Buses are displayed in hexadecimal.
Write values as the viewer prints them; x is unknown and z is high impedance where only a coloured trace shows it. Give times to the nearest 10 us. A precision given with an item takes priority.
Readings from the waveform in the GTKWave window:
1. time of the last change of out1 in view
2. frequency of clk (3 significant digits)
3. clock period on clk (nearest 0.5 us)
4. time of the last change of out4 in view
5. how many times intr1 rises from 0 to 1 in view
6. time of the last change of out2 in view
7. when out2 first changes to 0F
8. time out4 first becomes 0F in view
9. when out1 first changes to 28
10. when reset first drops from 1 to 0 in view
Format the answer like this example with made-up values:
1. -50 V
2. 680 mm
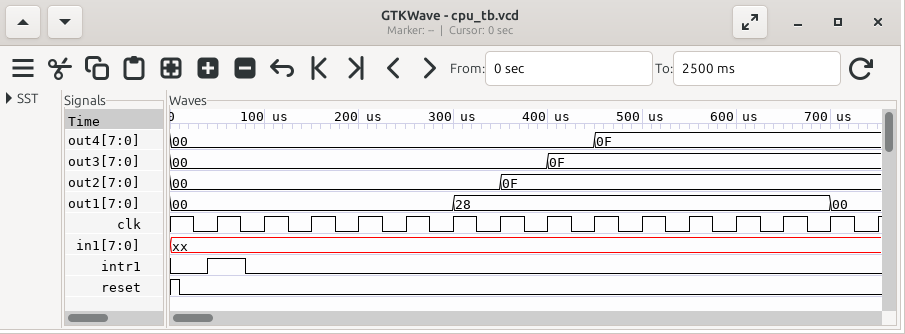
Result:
1. 700 us
2. 20.0 kHz
3. 50 us
4. 450 us
5. 1
6. 350 us
7. 350 us
8. 450 us
9. 300 us
10. 10 us
